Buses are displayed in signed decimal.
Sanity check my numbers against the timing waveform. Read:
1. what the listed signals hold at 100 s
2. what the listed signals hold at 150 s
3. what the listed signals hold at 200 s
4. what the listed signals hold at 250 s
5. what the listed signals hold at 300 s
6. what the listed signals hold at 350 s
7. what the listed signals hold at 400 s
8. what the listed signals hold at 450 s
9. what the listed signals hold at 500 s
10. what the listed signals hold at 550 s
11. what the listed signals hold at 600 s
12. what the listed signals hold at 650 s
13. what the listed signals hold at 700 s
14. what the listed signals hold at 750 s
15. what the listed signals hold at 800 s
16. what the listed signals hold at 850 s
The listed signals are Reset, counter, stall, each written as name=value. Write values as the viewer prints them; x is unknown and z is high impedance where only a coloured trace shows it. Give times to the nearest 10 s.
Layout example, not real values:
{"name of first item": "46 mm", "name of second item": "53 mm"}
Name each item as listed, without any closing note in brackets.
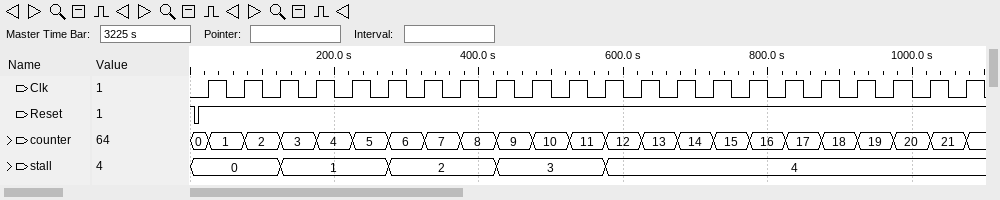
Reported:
{"what the listed signals hold at 100 s": "Reset=1, counter=2, stall=0", "what the listed signals hold at 150 s": "Reset=1, counter=3, stall=1", "what the listed signals hold at 200 s": "Reset=1, counter=4, stall=1", "what the listed signals hold at 250 s": "Reset=1, counter=5, stall=1", "what the listed signals hold at 300 s": "Reset=1, counter=6, stall=2", "what the listed signals hold at 350 s": "Reset=1, counter=7, stall=2", "what the listed signals hold at 400 s": "Reset=1, counter=8, stall=2", "what the listed signals hold at 450 s": "Reset=1, counter=9, stall=3", "what the listed signals hold at 500 s": "Reset=1, counter=10, stall=3", "what the listed signals hold at 550 s": "Reset=1, counter=11, stall=3", "what the listed signals hold at 600 s": "Reset=1, counter=12, stall=4", "what the listed signals hold at 650 s": "Reset=1, counter=13, stall=4", "what the listed signals hold at 700 s": "Reset=1, counter=14, stall=4", "what the listed signals hold at 750 s": "Reset=1, counter=15, stall=4", "what the listed signals hold at 800 s": "Reset=1, counter=16, stall=4", "what the listed signals hold at 850 s": "Reset=1, counter=17, stall=4"}
